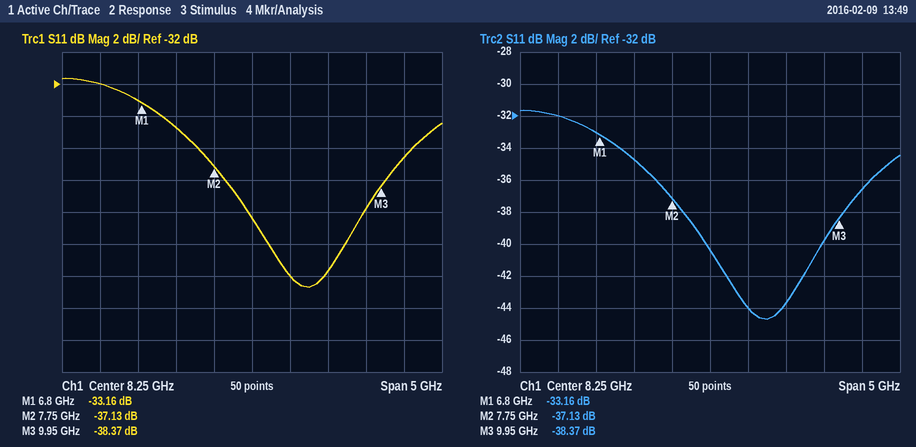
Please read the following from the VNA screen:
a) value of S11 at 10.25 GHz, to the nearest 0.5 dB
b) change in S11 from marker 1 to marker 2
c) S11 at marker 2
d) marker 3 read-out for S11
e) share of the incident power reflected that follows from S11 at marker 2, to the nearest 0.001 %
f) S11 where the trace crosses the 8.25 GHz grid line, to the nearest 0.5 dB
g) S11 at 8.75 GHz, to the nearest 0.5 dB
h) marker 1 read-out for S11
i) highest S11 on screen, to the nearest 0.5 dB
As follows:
-36.5 dB
-3.97 dB
-37.13 dB
-38.37 dB
0.019 %
-40.5 dB
-44.0 dB
-33.16 dB
-31.5 dB
